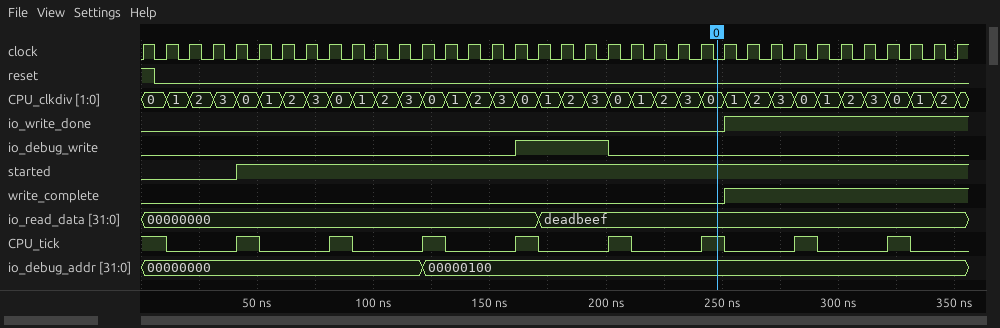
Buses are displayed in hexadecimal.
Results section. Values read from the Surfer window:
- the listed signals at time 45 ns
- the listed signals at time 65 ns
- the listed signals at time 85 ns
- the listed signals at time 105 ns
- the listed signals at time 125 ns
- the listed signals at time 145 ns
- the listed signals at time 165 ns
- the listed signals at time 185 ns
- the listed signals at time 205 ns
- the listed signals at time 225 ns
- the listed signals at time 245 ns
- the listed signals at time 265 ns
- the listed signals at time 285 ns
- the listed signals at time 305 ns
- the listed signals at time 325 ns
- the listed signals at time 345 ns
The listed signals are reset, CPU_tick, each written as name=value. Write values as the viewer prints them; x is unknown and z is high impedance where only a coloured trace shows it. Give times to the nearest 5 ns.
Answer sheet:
reset=0, CPU_tick=1
reset=0, CPU_tick=0
reset=0, CPU_tick=1
reset=0, CPU_tick=0
reset=0, CPU_tick=1
reset=0, CPU_tick=0
reset=0, CPU_tick=1
reset=0, CPU_tick=0
reset=0, CPU_tick=1
reset=0, CPU_tick=0
reset=0, CPU_tick=1
reset=0, CPU_tick=0
reset=0, CPU_tick=1
reset=0, CPU_tick=0
reset=0, CPU_tick=1
reset=0, CPU_tick=0
